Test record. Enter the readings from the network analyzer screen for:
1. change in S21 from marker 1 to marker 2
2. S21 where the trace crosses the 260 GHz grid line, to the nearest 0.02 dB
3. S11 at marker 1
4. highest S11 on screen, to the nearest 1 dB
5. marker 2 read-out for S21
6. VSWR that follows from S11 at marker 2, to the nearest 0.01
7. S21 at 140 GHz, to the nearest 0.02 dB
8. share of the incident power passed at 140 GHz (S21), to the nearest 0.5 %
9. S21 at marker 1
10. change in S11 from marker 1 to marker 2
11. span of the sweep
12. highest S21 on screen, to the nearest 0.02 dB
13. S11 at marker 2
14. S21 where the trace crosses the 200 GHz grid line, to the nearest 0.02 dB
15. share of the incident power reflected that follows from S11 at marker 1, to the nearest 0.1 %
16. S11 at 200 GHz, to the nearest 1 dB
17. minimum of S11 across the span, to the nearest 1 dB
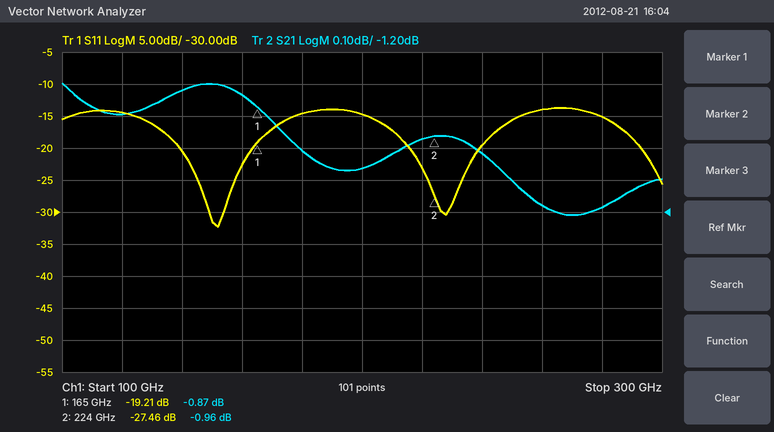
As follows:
-0.09 dB
-1.18 dB
-19.21 dB
-14 dB
-0.96 dB
1.09
-0.82 dB
83.0 %
-0.87 dB
-8.25 dB
200 GHz
-0.80 dB
-27.46 dB
-1.06 dB
1.2 %
-15 dB
-32 dB
